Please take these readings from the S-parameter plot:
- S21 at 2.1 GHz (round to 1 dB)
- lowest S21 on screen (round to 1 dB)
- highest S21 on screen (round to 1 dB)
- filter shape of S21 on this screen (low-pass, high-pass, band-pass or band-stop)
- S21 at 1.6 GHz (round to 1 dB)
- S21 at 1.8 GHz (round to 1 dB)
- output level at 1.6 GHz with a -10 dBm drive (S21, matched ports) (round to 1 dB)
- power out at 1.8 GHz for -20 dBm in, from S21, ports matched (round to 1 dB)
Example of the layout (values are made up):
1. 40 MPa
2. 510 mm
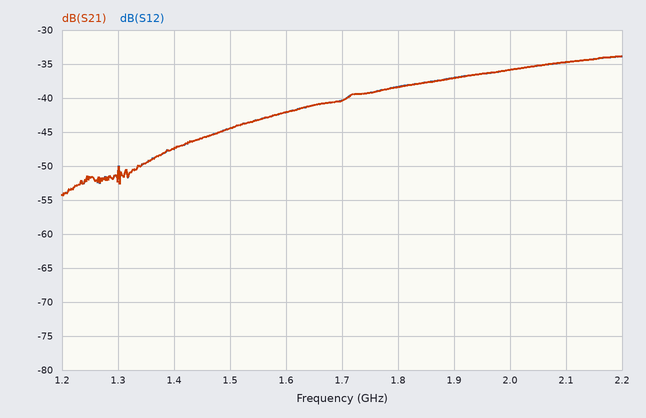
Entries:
1. -35 dB
2. -54 dB
3. -34 dB
4. high-pass
5. -42 dB
6. -38 dB
7. -52 dBm
8. -58 dBm
